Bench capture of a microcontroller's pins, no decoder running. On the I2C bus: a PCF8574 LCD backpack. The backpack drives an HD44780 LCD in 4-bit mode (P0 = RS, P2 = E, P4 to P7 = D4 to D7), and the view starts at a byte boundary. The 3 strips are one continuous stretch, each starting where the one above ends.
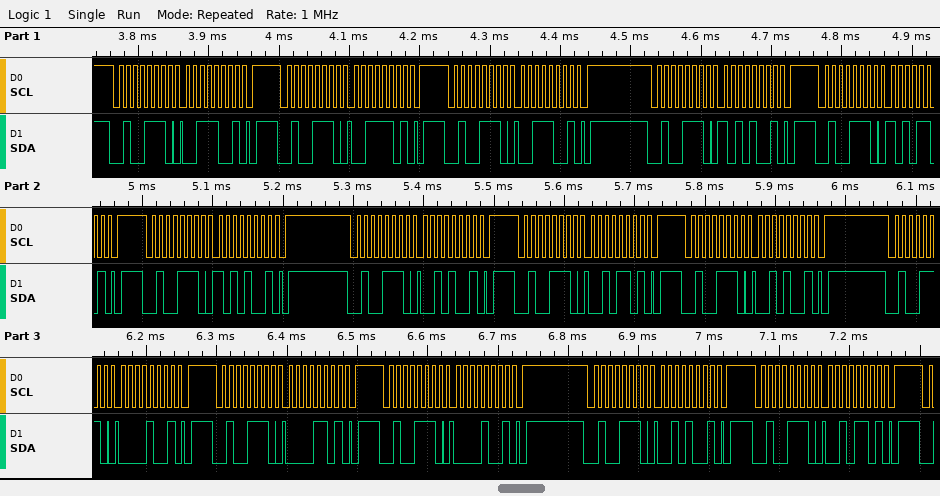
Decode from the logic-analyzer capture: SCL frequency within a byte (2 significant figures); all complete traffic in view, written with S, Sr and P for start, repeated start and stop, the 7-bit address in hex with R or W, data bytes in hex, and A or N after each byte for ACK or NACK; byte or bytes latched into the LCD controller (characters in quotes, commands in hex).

100 kHz
S 27W A 39 A P S 27W A 3D A P S 27W A 39 A P S 27W A A9 A P S 27W A AD A P S 27W A A9 A P S 27W A 29 A P S 27W A 2D A P S 27W A 29 A P S 27W A 09 A P S 27W A 0D A P S 27W A 09 A P S 27W A 29 A P S 27W A 2D A P
':' ' '
